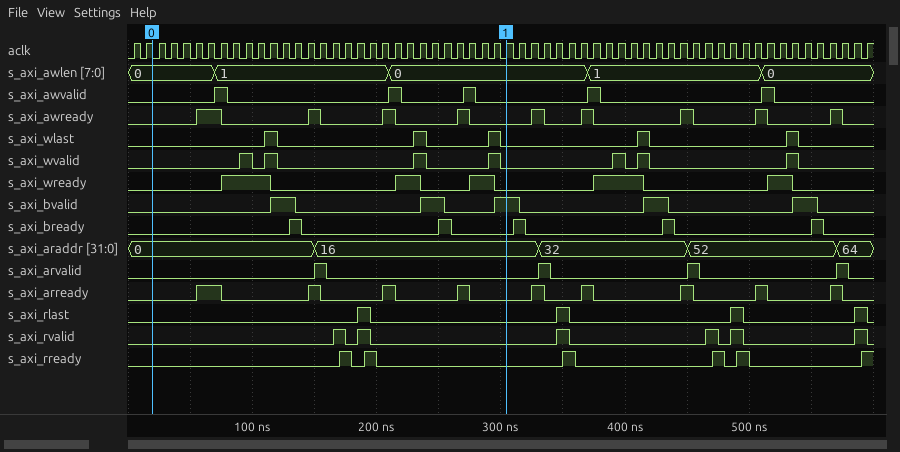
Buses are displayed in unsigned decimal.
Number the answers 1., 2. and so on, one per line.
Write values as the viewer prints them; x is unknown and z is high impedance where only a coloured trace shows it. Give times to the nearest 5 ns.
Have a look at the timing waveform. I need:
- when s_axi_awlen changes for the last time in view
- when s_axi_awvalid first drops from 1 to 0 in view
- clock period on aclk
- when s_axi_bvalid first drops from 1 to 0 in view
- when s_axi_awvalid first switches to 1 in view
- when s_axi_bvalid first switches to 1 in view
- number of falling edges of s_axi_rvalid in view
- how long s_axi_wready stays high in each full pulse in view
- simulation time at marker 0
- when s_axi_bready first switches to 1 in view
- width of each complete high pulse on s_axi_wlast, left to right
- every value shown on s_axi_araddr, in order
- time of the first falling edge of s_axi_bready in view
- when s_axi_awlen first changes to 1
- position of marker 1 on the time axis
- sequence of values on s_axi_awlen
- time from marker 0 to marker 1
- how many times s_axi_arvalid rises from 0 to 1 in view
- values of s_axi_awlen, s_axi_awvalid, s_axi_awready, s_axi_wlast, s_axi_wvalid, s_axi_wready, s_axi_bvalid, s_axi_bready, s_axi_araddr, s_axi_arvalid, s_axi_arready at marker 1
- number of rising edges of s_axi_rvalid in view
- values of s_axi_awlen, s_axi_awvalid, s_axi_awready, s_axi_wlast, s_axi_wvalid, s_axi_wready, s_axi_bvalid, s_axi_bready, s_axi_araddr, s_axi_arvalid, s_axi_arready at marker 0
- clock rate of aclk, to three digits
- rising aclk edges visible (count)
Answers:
1. 510 ns
2. 80 ns
3. 10 ns
4. 135 ns
5. 70 ns
6. 115 ns
7. 6
8. 40 ns, 20 ns, 20 ns, 40 ns, 20 ns
9. 20 ns
10. 130 ns
11. 10 ns, 10 ns, 10 ns, 10 ns, 10 ns
12. 0, 16, 32, 52, 64
13. 140 ns
14. 70 ns
15. 305 ns
16. 0, 1, 0, 1, 0
17. 285 ns
18. 4
19. s_axi_awlen=0, s_axi_awvalid=0, s_axi_awready=0, s_axi_wlast=0, s_axi_wvalid=0, s_axi_wready=0, s_axi_bvalid=1, s_axi_bready=0, s_axi_araddr=16, s_axi_arvalid=0, s_axi_arready=0
20. 6
21. s_axi_awlen=0, s_axi_awvalid=0, s_axi_awready=0, s_axi_wlast=0, s_axi_wvalid=0, s_axi_wready=0, s_axi_bvalid=0, s_axi_bready=0, s_axi_araddr=0, s_axi_arvalid=0, s_axi_arready=0
22. 100 MHz
23. 60
